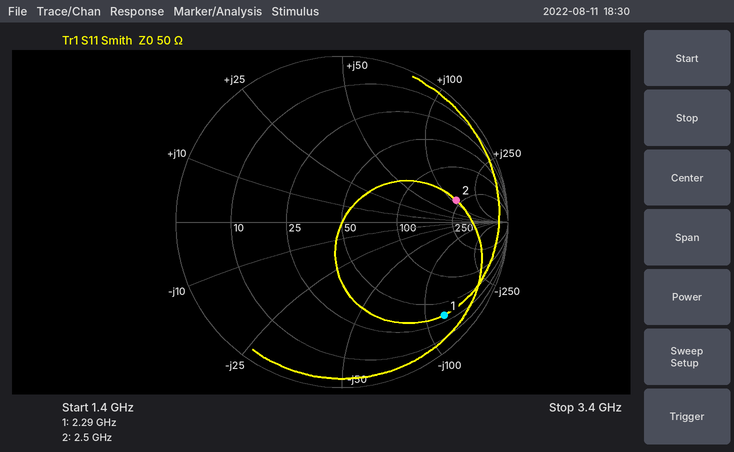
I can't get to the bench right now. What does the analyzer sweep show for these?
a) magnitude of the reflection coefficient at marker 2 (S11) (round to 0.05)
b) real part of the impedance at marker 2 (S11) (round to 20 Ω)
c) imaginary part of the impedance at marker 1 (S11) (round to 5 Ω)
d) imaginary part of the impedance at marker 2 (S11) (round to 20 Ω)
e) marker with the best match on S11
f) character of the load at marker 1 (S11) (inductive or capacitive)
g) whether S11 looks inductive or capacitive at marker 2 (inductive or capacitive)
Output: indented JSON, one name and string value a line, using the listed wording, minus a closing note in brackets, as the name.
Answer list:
{
  "magnitude of the reflection coefficient at marker 2 (S11)": "0.70",
  "real part of the impedance at marker 2 (S11)": "220 Ω",
  "imaginary part of the impedance at marker 1 (S11)": "-120 Ω",
  "imaginary part of the impedance at marker 2 (S11)": "+120 Ω",
  "marker with the best match on S11": "marker 2",
  "character of the load at marker 1 (S11)": "capacitive",
  "whether S11 looks inductive or capacitive at marker 2": "inductive"
}
